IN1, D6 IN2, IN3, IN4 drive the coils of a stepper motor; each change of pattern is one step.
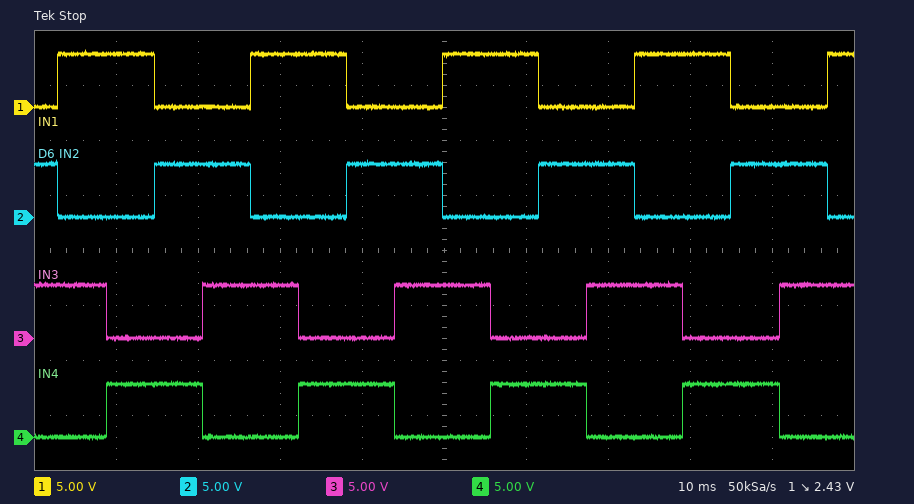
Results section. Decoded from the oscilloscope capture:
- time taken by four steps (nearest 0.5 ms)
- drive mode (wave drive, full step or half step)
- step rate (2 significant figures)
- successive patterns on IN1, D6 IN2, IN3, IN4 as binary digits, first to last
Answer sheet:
23.5 ms
full step
170 steps/s
0110 1010 1001 0101 0110 1010 1001 0101 0110 1010 1001 0101 0110 1010 1001 0101 0110 1010
